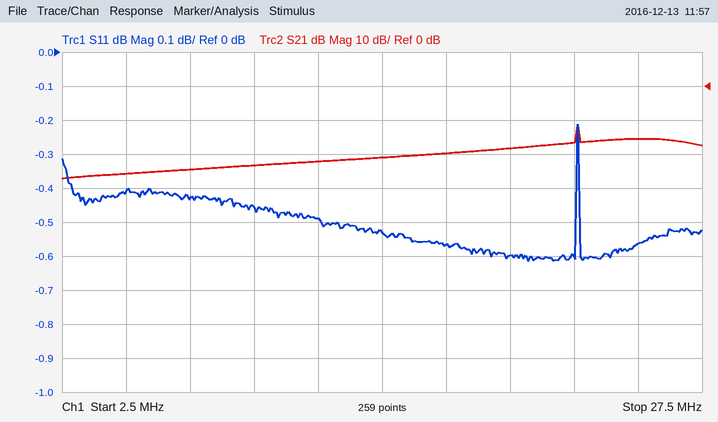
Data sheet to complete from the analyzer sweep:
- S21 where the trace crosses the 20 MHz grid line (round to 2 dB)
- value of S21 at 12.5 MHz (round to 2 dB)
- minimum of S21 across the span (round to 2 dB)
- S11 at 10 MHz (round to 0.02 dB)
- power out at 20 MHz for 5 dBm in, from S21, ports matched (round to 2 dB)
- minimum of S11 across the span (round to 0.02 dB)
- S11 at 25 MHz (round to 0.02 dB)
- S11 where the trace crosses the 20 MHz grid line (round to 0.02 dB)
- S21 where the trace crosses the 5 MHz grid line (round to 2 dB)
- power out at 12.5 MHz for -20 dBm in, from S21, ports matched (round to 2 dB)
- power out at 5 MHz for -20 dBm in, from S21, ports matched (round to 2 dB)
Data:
-18 dB
-22 dB
-28 dB
-0.46 dB
-14 dBm
-0.62 dB
-0.56 dB
-0.60 dB
-26 dB
-42 dBm
-46 dBm
